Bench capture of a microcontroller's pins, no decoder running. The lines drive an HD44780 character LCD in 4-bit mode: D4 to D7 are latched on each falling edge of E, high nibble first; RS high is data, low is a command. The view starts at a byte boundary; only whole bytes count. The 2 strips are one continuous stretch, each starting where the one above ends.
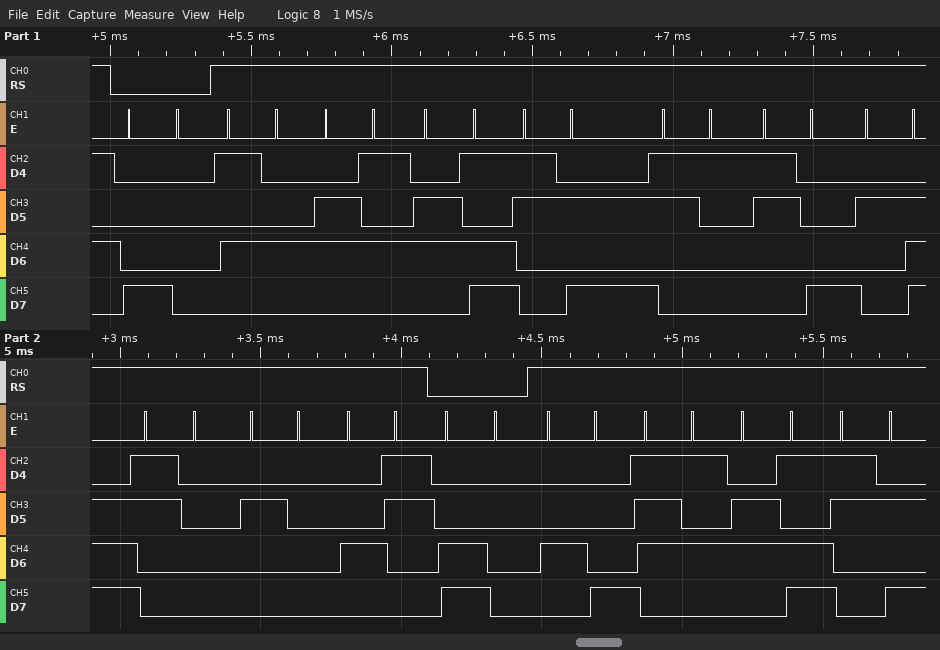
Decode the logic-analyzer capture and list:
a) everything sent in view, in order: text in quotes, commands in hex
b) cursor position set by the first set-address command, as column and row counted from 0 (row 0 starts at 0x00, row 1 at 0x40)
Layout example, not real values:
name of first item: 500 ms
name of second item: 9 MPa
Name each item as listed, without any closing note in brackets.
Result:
everything sent in view, in order: text in quotes, commands in hex: 0x80 "Tem:18.0 C" 0xC0 "Hum:"
cursor position set by the first set-address command, as column and row counted from 0: column 0, row 0
